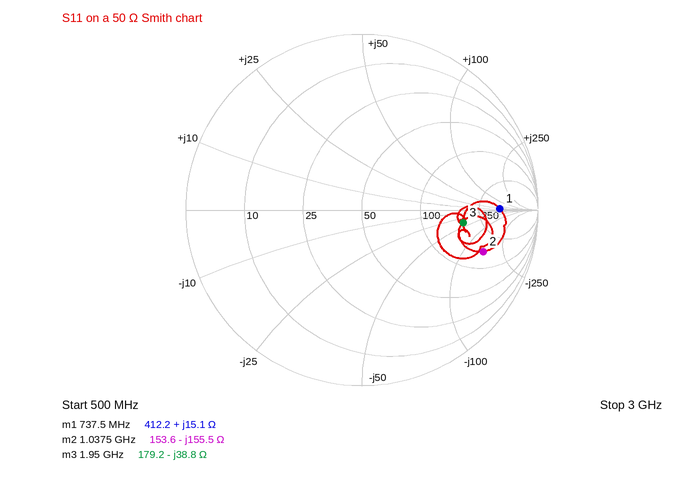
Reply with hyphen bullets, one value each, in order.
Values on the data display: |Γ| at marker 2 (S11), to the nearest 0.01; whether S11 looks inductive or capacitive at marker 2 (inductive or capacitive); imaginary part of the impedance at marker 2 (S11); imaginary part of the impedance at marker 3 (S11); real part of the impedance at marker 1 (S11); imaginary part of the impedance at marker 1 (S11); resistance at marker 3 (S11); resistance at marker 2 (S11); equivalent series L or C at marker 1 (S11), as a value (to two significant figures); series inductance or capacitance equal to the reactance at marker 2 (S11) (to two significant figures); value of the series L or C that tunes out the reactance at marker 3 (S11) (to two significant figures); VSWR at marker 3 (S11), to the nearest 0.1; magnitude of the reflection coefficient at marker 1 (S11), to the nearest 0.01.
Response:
- 0.73
- capacitive
- -155.5 Ω
- -38.8 Ω
- 412.2 Ω
- +15.1 Ω
- 179.2 Ω
- 153.6 Ω
- 3.3 nH
- 990 fF
- 3.2 nH
- 3.8
- 0.78
